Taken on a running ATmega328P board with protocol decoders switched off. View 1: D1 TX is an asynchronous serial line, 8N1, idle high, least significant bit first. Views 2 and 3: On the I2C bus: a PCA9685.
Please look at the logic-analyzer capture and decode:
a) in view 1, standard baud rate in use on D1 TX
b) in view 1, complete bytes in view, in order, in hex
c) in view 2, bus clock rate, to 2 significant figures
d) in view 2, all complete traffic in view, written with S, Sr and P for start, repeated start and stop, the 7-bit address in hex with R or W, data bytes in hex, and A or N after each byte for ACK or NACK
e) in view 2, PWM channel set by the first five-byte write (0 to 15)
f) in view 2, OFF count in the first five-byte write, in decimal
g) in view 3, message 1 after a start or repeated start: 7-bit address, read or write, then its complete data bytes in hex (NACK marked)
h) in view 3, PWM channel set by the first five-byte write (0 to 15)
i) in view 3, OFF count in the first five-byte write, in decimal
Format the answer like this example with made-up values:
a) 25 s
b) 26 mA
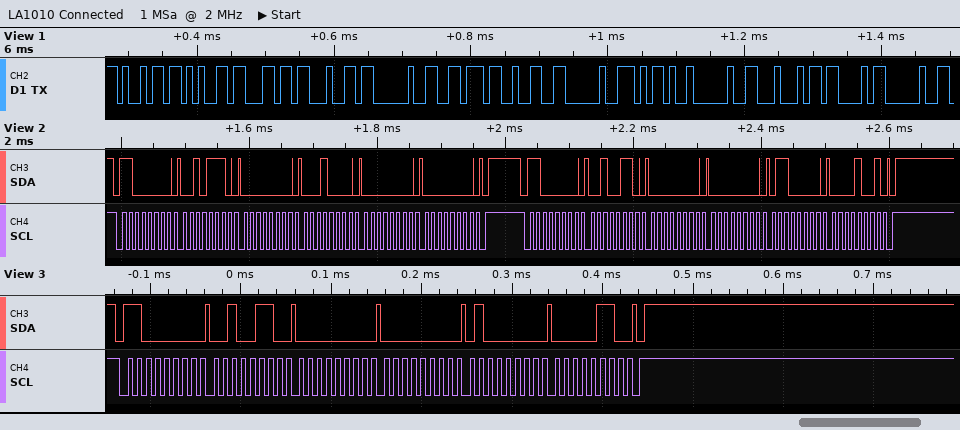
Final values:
a) 115200 baud
b) 69 65 6C 64 20 76 32 20 2D 20 44 43 20
c) 100 kHz
d) S 60W A 2E A 00 A 10 A 00 A 00 A P S 60W A 26 A 00 A 00 A 60 A 09 A P
e) 10
f) 0
g) 0x60 write: 26 00 00 40 06
h) 8
i) 1600
